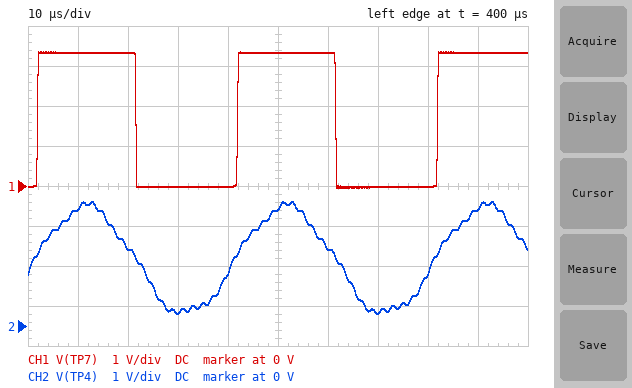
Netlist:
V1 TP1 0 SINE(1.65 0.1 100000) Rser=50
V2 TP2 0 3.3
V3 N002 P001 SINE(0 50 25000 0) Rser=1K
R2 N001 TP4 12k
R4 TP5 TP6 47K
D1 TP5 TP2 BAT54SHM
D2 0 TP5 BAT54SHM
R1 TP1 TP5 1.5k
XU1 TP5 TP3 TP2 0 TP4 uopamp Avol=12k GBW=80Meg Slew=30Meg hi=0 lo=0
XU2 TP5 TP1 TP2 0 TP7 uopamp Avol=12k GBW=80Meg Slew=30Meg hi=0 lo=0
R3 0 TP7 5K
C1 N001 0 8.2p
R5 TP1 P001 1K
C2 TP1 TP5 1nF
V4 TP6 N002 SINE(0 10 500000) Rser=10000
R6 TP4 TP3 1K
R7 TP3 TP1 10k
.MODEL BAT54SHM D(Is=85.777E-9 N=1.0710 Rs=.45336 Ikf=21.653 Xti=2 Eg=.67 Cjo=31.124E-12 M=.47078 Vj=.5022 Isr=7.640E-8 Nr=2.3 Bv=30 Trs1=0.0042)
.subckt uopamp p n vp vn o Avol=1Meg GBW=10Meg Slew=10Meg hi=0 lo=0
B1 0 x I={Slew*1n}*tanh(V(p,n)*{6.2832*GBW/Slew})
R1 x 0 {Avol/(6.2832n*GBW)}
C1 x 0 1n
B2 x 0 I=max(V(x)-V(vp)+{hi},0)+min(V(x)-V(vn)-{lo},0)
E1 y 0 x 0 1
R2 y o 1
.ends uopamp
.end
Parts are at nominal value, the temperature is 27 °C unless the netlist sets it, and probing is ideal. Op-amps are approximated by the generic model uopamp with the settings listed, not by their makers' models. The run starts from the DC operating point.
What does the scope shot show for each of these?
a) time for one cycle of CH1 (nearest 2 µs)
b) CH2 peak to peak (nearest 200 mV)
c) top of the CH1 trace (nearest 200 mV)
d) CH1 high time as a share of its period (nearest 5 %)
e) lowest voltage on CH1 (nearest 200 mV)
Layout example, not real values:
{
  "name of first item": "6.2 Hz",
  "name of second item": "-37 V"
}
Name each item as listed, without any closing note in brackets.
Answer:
{
  "time for one cycle of CH1": "40 µs",
  "CH2 peak to peak": "2.8 V",
  "top of the CH1 trace": "3.4 V",
  "CH1 high time as a share of its period": "50 %",
  "lowest voltage on CH1": "0 V"
}
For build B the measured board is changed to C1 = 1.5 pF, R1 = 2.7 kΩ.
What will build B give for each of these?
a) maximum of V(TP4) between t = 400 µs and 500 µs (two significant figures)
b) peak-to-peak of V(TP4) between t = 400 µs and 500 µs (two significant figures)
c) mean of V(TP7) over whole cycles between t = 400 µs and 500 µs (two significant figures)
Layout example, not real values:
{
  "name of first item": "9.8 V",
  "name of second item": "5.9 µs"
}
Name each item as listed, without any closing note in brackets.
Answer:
{
  "maximum of V(TP4) between t = 400 µs and 500 µs": "3.3 V",
  "peak-to-peak of V(TP4) between t = 400 µs and 500 µs": "3.4 V",
  "mean of V(TP7) over whole cycles between t = 400 µs and 500 µs": "1.7 V"
}
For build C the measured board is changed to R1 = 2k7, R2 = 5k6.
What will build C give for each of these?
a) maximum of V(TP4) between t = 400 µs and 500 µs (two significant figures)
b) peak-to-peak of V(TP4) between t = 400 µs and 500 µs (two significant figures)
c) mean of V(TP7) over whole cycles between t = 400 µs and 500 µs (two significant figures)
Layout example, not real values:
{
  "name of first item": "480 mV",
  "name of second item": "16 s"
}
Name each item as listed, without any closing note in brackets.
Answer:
{
  "maximum of V(TP4) between t = 400 µs and 500 µs": "3.3 V",
  "peak-to-peak of V(TP4) between t = 400 µs and 500 µs": "3.4 V",
  "mean of V(TP7) over whole cycles between t = 400 µs and 500 µs": "1.7 V"
}
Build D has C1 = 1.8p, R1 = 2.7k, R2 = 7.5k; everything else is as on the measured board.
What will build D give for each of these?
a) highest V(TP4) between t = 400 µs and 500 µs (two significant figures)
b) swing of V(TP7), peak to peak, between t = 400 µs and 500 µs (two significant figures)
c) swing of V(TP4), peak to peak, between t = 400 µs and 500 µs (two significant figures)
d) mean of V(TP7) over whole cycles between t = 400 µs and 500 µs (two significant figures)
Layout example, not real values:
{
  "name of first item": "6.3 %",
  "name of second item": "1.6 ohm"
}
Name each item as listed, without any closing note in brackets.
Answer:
{
  "highest V(TP4) between t = 400 µs and 500 µs": "3.3 V",
  "swing of V(TP7), peak to peak, between t = 400 µs and 500 µs": "3.4 V",
  "swing of V(TP4), peak to peak, between t = 400 µs and 500 µs": "3.4 V",
  "mean of V(TP7) over whole cycles between t = 400 µs and 500 µs": "1.7 V"
}
